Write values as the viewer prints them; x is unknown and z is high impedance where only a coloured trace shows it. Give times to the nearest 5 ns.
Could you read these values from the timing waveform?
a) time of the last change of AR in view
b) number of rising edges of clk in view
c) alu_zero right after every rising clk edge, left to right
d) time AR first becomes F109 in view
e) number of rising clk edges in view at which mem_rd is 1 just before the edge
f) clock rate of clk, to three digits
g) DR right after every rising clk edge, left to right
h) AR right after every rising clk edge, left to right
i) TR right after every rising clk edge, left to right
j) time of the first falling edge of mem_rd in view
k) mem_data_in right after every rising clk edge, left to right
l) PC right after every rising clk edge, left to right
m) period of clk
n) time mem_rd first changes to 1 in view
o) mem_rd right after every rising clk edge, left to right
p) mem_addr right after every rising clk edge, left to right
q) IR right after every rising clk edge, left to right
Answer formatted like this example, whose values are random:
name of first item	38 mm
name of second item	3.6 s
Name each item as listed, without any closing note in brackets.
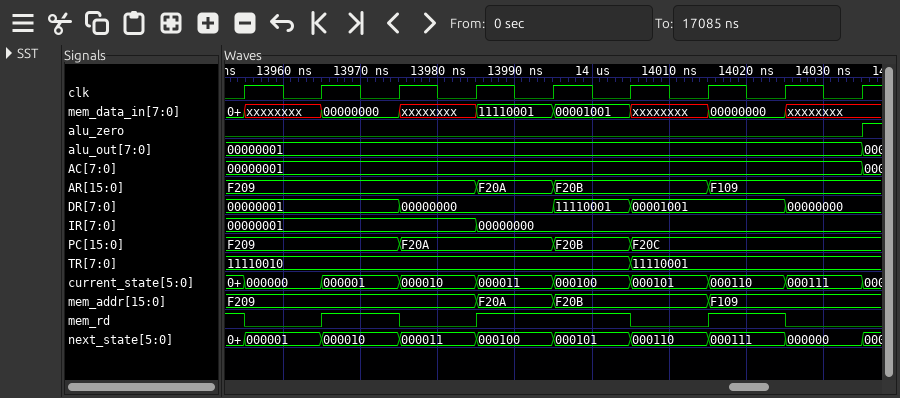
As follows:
time of the last change of AR in view	14015 ns
number of rising edges of clk in view	9
alu_zero right after every rising clk edge, left to right	0 0 0 0 0 0 0 0 1
time AR first becomes F109 in view	14015 ns
number of rising clk edges in view at which mem_rd is 1 just before the edge	5
clock rate of clk, to three digits	100 MHz
DR right after every rising clk edge, left to right	00000001, 00000001, 00000000, 00000000, 11110001, 00001001, 00001001, 00000000, 00000000
AR right after every rising clk edge, left to right	F209, F209, F209, F20A, F20B, F20B, F109, F109, F109
TR right after every rising clk edge, left to right	11110010, 11110010, 11110010, 11110010, 11110010, 11110001, 11110001, 11110001, 11110001
time of the first falling edge of mem_rd in view	13955 ns
mem_data_in right after every rising clk edge, left to right	xxxxxxxx, 00000000, xxxxxxxx, 11110001, 00001001, xxxxxxxx, 00000000, xxxxxxxx, xxxxxxxx
PC right after every rising clk edge, left to right	F209, F209, F20A, F20A, F20B, F20C, F20C, F20C, F20C
period of clk	10 ns
time mem_rd first changes to 1 in view	13965 ns
mem_rd right after every rising clk edge, left to right	0 1 0 1 1 0 1 0 0
mem_addr right after every rising clk edge, left to right	F209, F209, F209, F20A, F20B, F20B, F109, F109, F109
IR right after every rising clk edge, left to right	00000001, 00000001, 00000001, 00000000, 00000000, 00000000, 00000000, 00000000, 00000000
